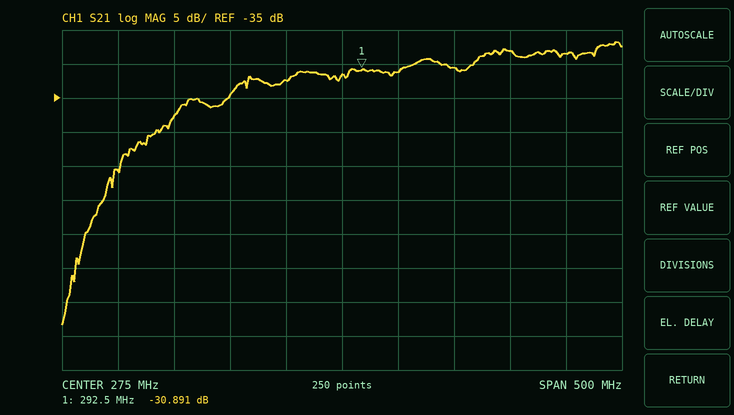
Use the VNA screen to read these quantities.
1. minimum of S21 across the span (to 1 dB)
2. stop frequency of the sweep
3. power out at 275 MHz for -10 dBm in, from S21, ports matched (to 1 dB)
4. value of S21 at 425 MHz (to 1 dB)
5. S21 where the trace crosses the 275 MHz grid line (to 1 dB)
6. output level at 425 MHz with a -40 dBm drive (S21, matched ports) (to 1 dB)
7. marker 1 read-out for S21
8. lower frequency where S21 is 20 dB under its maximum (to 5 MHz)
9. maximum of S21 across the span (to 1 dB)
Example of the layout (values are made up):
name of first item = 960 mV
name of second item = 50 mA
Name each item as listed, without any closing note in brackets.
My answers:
minimum of S21 across the span = -68 dB
stop frequency of the sweep = 525 MHz
power out at 275 MHz for -10 dBm in, from S21, ports matched = -42 dBm
value of S21 at 425 MHz = -28 dB
S21 where the trace crosses the 275 MHz grid line = -32 dB
output level at 425 MHz with a -40 dBm drive (S21, matched ports) = -68 dBm
marker 1 read-out for S21 = -30.891 dB
lower frequency where S21 is 20 dB under its maximum = 70 MHz
maximum of S21 across the span = -27 dB
